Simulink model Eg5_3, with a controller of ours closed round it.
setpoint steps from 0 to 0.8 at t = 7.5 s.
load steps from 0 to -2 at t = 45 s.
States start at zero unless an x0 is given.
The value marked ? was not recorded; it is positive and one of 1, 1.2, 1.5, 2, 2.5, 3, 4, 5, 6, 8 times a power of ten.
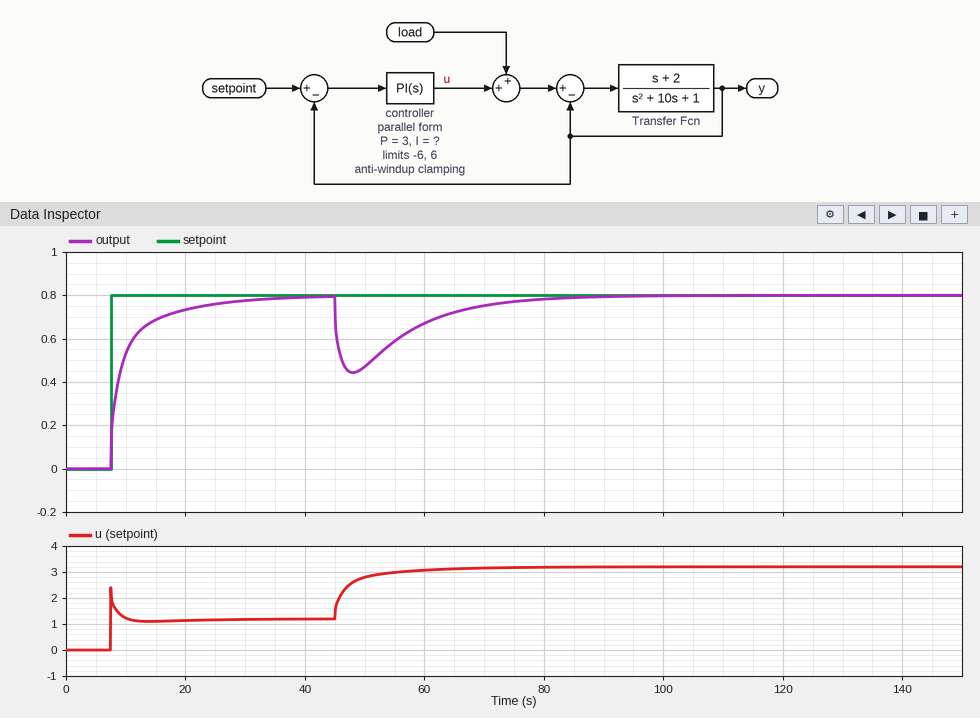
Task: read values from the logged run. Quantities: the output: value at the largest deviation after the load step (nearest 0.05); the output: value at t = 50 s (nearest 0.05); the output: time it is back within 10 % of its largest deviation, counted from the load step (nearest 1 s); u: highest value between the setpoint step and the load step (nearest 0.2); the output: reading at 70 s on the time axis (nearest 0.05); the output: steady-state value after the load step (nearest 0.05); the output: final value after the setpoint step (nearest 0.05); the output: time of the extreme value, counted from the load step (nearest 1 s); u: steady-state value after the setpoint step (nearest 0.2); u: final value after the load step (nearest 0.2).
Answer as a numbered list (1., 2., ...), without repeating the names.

1. 0.45
2. 0.45
3. 28 s
4. 2.4
5. 0.75
6. 0.80
7. 0.80
8. 3 s
9. 1.2
10. 3.2
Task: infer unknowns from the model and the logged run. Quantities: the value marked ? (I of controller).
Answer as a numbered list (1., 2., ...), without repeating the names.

1. 0.4
